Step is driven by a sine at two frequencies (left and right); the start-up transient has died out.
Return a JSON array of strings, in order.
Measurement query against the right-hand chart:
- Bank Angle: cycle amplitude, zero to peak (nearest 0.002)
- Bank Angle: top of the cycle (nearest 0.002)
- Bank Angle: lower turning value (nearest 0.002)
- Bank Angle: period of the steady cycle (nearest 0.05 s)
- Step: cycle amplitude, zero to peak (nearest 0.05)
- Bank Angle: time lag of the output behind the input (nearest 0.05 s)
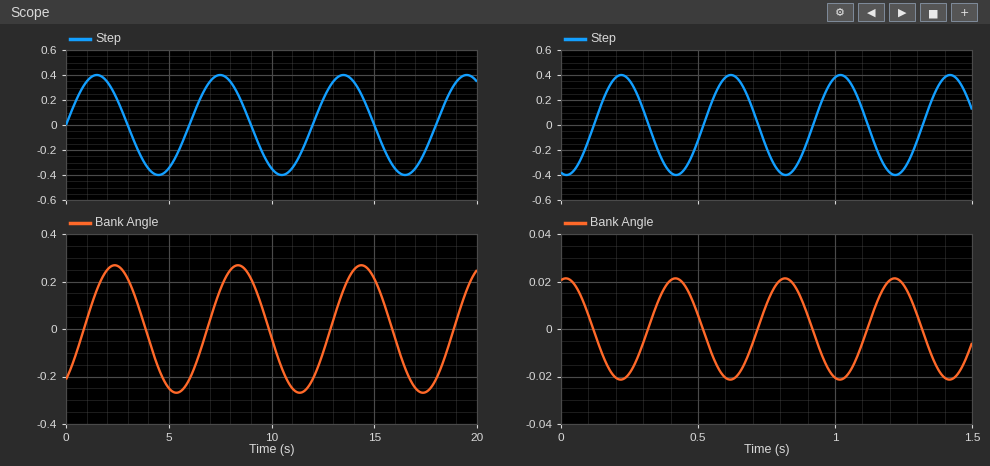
["0.022", "0.022", "-0.022", "0.40 s", "0.40", "0.20 s"]
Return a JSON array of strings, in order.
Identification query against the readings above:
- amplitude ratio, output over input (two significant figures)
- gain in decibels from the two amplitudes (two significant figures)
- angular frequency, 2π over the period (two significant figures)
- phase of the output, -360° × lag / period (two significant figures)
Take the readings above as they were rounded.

["0.055", "-25 dB", "16 rad/s", "-180°"]
